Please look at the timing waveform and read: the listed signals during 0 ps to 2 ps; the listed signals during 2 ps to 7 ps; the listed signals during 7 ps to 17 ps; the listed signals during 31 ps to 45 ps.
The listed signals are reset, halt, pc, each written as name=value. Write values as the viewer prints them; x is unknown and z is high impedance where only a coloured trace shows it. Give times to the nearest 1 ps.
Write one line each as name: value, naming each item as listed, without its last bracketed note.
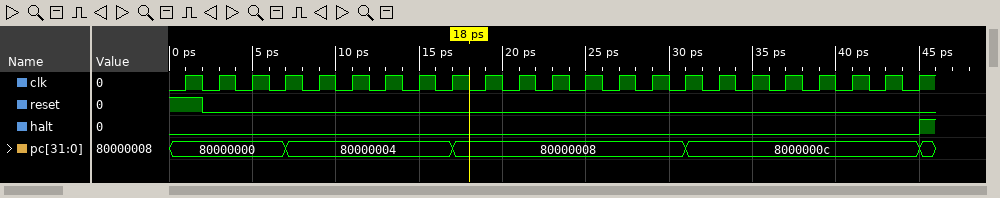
the listed signals during 0 ps to 2 ps: reset=1, halt=0, pc=80000000
the listed signals during 2 ps to 7 ps: reset=0, halt=0, pc=80000000
the listed signals during 7 ps to 17 ps: reset=0, halt=0, pc=80000004
the listed signals during 31 ps to 45 ps: reset=0, halt=0, pc=8000000c
